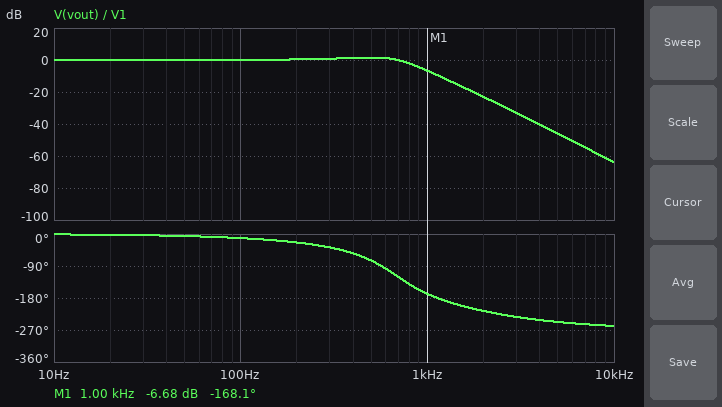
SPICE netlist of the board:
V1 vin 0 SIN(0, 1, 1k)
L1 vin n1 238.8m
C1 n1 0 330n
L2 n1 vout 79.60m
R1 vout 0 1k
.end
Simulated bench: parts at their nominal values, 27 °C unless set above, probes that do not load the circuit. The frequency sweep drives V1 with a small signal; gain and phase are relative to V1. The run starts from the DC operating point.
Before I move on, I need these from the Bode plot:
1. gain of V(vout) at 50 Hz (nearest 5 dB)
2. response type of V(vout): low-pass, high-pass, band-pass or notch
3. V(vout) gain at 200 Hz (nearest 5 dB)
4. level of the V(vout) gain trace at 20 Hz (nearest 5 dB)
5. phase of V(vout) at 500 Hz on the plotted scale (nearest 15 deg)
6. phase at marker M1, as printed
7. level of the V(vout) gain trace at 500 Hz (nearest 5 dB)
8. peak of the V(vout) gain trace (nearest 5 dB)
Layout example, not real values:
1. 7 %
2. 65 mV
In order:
1. 0 dB
2. low-pass
3. 0 dB
4. 0 dB
5. -75 deg
6. -168.1 deg
7. 0 dB
8. 0 dB
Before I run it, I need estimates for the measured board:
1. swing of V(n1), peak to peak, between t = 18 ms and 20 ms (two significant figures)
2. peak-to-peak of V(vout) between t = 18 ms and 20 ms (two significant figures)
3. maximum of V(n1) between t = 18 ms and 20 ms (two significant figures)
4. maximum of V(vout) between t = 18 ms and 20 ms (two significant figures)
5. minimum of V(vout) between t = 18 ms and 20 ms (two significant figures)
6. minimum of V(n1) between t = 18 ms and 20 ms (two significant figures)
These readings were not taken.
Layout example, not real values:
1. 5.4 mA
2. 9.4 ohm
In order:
1. 1.0 V
2. 930 mV
3. 520 mV
4. 460 mV
5. -460 mV
6. -520 mV
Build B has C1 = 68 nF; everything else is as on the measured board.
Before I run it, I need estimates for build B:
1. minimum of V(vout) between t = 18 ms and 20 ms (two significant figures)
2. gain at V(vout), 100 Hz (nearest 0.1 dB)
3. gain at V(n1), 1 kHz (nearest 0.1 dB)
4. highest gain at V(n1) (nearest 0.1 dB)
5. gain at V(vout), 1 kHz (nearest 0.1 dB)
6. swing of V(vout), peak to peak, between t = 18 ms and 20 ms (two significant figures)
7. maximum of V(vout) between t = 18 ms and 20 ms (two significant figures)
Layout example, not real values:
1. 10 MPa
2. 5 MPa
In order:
1. -580 mV
2. -0.1 dB
3. -3.7 dB
4. 0 dB
5. -4.7 dB
6. 1.2 V
7. 580 mV
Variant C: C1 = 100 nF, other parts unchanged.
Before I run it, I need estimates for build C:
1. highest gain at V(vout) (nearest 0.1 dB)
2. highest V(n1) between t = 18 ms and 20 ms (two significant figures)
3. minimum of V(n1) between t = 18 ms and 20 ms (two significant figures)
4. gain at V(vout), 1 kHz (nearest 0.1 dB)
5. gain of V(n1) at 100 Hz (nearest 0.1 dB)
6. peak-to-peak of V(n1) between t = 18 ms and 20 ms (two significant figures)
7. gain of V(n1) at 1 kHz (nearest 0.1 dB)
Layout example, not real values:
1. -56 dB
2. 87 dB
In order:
1. 0 dB
2. 730 mV
3. -730 mV
4. -3.7 dB
5. -0.1 dB
6. 1.5 V
7. -2.7 dB
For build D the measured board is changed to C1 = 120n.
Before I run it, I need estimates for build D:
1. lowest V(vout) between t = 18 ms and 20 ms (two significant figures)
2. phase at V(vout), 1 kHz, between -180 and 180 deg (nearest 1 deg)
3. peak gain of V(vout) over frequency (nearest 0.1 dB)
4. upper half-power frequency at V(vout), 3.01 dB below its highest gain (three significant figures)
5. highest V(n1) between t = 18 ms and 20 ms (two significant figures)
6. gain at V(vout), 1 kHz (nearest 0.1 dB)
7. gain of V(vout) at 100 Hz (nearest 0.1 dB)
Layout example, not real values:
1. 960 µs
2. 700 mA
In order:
1. -690 mV
2. -95 deg
3. 0 dB
4. 947 Hz
5. 780 mV
6. -3.2 dB
7. -0.1 dB
